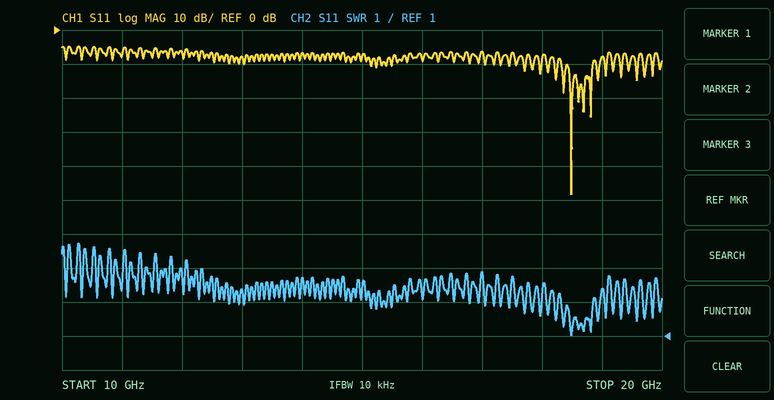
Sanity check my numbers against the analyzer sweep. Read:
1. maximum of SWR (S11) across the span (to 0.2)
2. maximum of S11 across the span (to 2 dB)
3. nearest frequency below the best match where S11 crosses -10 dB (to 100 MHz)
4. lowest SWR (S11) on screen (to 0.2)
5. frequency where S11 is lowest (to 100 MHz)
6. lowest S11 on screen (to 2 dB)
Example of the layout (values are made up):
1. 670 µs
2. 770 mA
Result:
1. 3.8
2. -4 dB
3. 18.3 GHz
4. 1.0
5. 18.5 GHz
6. -48 dB
